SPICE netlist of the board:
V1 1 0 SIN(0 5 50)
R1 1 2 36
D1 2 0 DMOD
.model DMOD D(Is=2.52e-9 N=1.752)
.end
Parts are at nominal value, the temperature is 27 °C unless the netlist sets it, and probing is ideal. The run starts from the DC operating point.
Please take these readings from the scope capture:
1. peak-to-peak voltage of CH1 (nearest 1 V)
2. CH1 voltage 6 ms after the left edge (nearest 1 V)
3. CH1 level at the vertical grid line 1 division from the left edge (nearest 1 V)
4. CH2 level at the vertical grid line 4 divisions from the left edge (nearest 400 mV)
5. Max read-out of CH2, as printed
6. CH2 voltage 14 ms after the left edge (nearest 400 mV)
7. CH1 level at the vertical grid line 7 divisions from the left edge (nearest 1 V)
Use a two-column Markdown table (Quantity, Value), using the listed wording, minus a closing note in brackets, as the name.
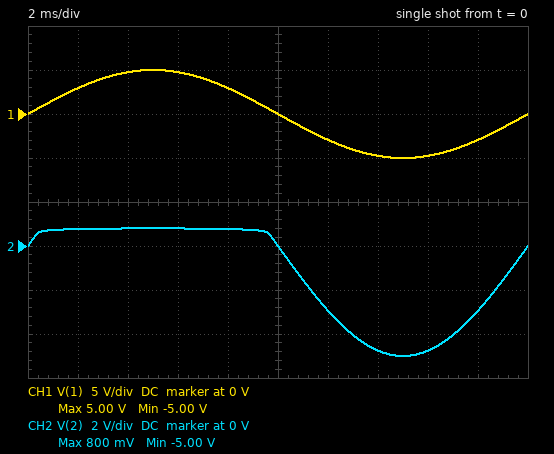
| Quantity | Value |
|---|---|
| peak-to-peak voltage of CH1 | 10 V |
| CH1 voltage 6 ms after the left edge | 5 V |
| CH1 level at the vertical grid line 1 division from the left edge | 3 V |
| CH2 level at the vertical grid line 4 divisions from the left edge | 800 mV |
| Max read-out of CH2, as printed | 800 mV |
| CH2 voltage 14 ms after the left edge | -4.8 V |
| CH1 level at the vertical grid line 7 divisions from the left edge | -5 V |
